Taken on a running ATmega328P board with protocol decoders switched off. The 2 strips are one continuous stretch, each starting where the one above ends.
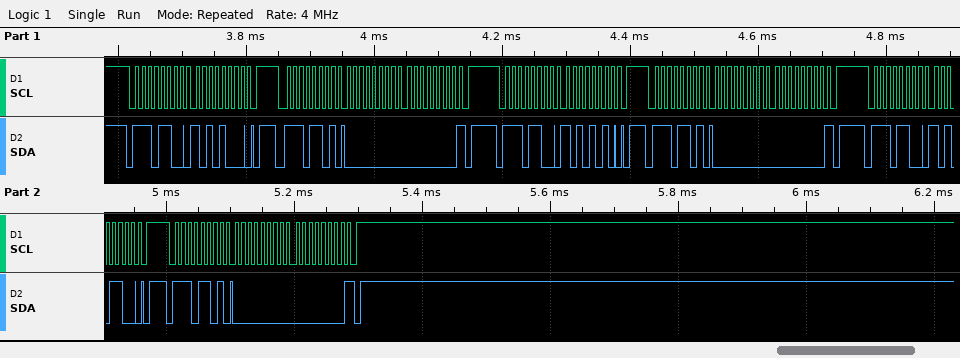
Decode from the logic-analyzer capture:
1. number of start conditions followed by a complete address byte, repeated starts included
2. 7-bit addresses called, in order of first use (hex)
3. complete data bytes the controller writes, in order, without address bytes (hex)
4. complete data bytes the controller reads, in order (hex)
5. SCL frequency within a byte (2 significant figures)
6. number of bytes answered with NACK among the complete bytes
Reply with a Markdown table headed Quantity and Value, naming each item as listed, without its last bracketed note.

| Quantity | Value |
|---|---|
| number of start conditions followed by a complete address byte, repeated starts included | 6 |
| 7-bit addresses called, in order of first use | 0x76 |
| complete data bytes the controller writes, in order, without address bytes | A8 AA AC |
| complete data bytes the controller reads, in order | 00 00 00 00 00 00 |
| SCL frequency within a byte | 100 kHz |
| number of bytes answered with NACK among the complete bytes | 3 |
